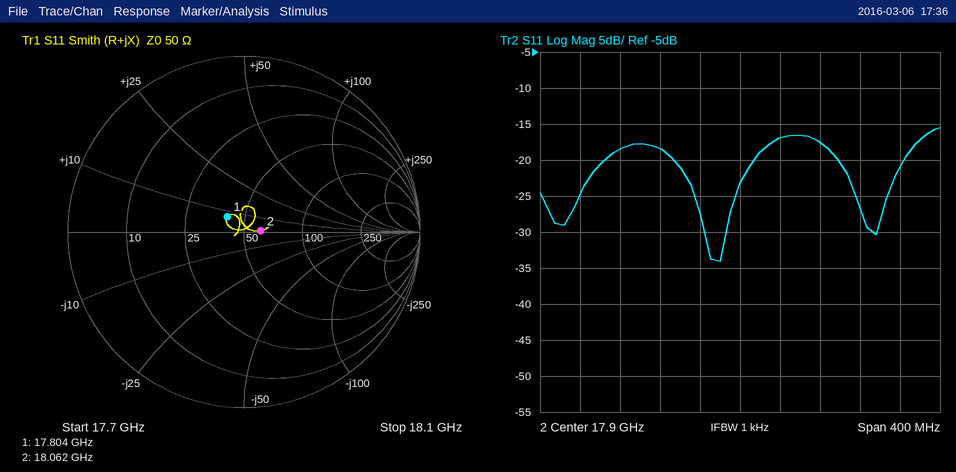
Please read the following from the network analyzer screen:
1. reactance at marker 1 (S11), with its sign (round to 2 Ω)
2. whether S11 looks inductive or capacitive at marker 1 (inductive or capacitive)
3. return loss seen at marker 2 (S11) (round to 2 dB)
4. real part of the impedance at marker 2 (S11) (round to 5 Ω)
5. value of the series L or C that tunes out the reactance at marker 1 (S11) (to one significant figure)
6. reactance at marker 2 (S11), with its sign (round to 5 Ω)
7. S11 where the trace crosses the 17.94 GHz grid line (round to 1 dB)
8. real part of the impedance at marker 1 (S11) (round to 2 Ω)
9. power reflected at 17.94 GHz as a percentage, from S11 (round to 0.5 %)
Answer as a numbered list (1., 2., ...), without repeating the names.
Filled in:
1. +8 Ω
2. inductive
3. 20 dB
4. 60 Ω
5. 1 pF
6. 0 Ω
7. -17 dB
8. 40 Ω
9. 2.0 %
